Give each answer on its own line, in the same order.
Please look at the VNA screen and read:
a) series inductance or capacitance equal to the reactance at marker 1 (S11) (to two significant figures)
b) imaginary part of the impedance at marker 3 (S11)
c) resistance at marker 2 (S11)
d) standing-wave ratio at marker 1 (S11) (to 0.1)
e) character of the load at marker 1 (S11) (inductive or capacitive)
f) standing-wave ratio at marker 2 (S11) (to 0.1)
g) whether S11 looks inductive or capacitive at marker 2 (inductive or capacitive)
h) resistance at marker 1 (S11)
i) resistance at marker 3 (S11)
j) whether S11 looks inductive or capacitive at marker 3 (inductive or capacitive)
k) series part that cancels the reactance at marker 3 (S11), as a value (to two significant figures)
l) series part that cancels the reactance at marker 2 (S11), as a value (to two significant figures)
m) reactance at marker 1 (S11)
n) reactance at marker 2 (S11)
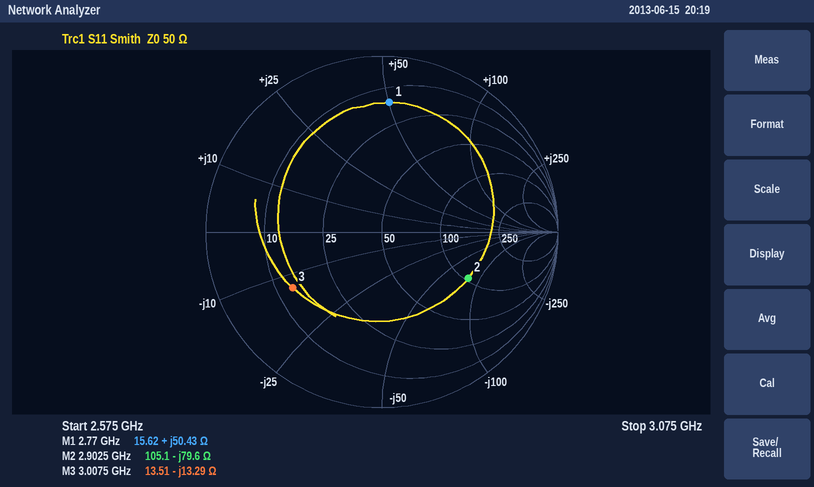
2.9 nH
-13.29 Ω
105.1 Ω
6.6
inductive
3.5
capacitive
15.62 Ω
13.51 Ω
capacitive
700 pH
4.4 nH
+50.43 Ω
-79.6 Ω
